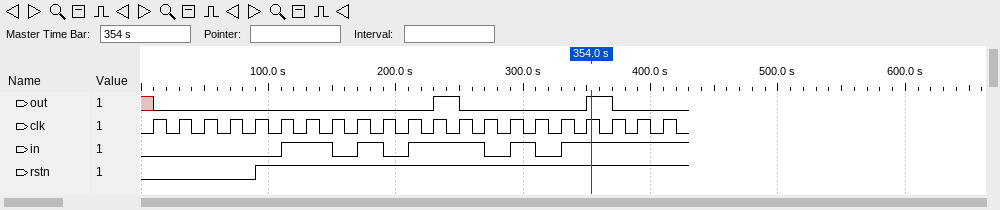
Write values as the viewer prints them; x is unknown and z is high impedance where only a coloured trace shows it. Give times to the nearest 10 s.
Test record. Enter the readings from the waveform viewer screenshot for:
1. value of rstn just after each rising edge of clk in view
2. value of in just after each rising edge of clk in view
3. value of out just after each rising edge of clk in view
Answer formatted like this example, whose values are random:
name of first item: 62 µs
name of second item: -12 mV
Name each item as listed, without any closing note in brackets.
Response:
value of rstn just after each rising edge of clk in view: 0 0 0 0 1 1 1 1 1 1 1 1 1 1 1 1 1 1 1 1 1
value of in just after each rising edge of clk in view: 0 0 0 0 0 1 1 0 1 0 1 1 1 0 1 0 1 1 1 1 1
value of out just after each rising edge of clk in view: 0 0 0 0 0 0 0 0 0 0 0 1 0 0 0 0 0 1 0 0 0
